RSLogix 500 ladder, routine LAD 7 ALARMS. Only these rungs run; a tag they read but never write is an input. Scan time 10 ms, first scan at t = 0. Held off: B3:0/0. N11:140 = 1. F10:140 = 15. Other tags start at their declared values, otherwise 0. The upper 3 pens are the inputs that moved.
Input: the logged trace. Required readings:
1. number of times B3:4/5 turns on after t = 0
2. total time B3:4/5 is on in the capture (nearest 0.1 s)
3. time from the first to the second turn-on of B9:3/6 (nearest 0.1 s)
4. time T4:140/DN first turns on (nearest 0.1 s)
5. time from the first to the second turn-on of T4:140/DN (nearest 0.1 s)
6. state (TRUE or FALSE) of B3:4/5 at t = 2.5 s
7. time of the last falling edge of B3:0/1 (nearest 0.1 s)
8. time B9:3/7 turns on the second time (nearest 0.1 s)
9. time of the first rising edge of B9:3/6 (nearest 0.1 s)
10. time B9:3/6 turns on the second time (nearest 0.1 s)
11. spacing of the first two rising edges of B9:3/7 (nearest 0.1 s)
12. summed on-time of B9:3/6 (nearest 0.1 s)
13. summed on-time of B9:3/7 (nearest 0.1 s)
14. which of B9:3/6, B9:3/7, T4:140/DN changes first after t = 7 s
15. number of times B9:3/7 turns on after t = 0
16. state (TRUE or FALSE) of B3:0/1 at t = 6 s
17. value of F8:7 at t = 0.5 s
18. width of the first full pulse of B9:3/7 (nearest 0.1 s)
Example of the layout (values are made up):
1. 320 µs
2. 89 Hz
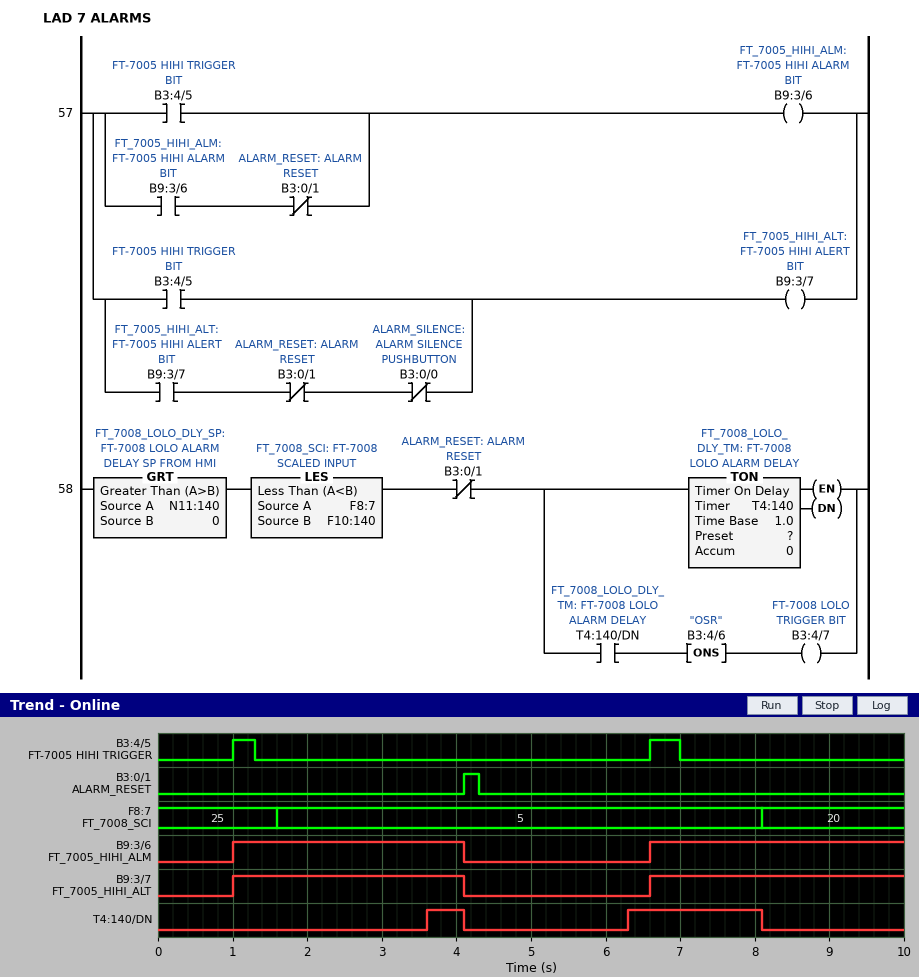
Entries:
1. 2
2. 0.7 s
3. 5.6 s
4. 3.6 s
5. 2.7 s
6. FALSE
7. 4.3 s
8. 6.6 s
9. 1.0 s
10. 6.6 s
11. 5.6 s
12. 6.5 s
13. 6.5 s
14. T4:140/DN
15. 2
16. FALSE
17. 25
18. 3.1 s
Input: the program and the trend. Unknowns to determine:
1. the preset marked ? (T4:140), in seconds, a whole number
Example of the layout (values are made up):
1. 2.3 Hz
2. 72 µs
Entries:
1. 2 s
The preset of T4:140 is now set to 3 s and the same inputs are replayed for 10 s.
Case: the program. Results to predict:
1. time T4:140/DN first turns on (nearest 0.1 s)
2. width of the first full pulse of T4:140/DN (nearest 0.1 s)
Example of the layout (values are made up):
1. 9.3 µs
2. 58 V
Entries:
1. 7.3 s
2. 0.8 s
